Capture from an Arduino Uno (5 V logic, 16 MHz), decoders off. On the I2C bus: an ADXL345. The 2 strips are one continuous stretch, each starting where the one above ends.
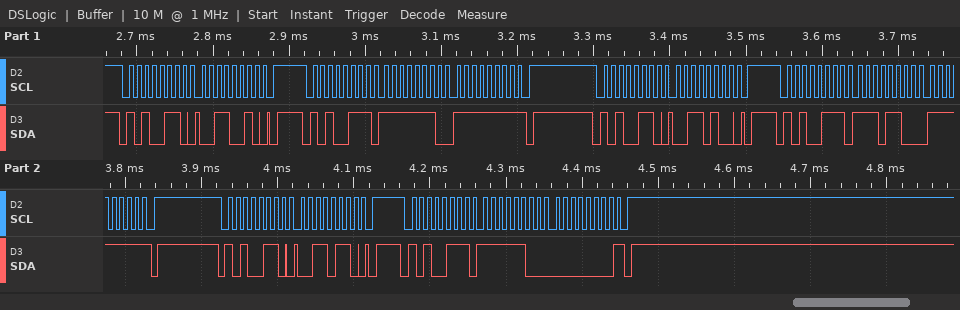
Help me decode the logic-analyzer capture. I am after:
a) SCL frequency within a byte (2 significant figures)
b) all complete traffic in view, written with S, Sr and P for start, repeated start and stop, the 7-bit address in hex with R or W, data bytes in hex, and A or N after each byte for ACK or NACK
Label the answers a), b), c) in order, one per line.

a) 100 kHz
b) S 53W A 32 A P S 53R A FE A FF N P S 53W A 34 A P S 53R A EC A FF N P S 53W A 36 A P S 53R A FC A 00 N P
